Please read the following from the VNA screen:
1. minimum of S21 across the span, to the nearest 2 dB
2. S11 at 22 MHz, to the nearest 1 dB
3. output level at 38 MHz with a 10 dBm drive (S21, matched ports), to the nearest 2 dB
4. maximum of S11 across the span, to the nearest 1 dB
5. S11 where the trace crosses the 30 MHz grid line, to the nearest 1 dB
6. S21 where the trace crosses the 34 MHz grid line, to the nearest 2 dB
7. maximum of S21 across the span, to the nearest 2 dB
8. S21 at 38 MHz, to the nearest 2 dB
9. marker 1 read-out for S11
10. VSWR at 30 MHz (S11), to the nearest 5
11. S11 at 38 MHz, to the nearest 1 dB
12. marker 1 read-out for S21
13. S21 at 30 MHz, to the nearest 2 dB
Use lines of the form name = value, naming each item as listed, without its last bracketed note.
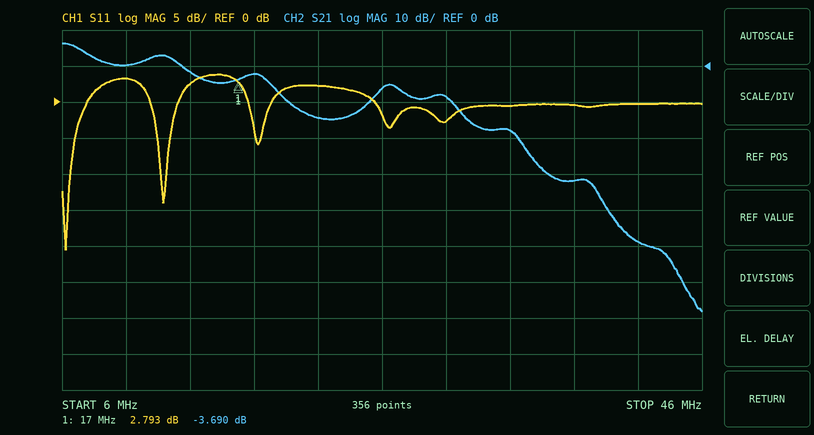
minimum of S21 across the span, to the nearest 2 dB = -68 dB
S11 at 22 MHz, to the nearest 1 dB = 2 dB
output level at 38 MHz with a 10 dBm drive (S21, matched ports), to the nearest 2 dB = -22 dBm
maximum of S11 across the span, to the nearest 1 dB = 4 dB
S11 where the trace crosses the 30 MHz grid line, to the nearest 1 dB = -3 dB
S21 where the trace crosses the 34 MHz grid line, to the nearest 2 dB = -18 dB
maximum of S21 across the span, to the nearest 2 dB = 6 dB
S21 at 38 MHz, to the nearest 2 dB = -32 dB
marker 1 read-out for S11 = 2.793 dB
VSWR at 30 MHz (S11), to the nearest 5 = 5
S11 at 38 MHz, to the nearest 1 dB = 0 dB
marker 1 read-out for S21 = -3.690 dB
S21 at 30 MHz, to the nearest 2 dB = -8 dB
